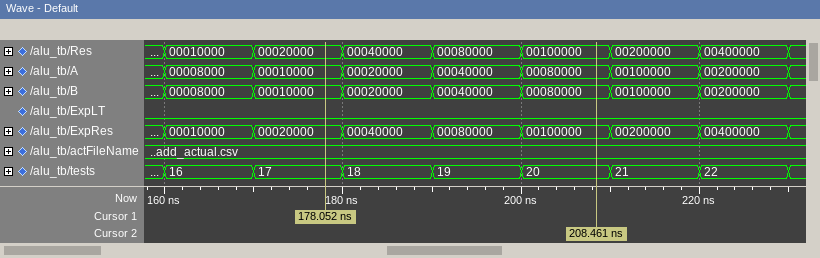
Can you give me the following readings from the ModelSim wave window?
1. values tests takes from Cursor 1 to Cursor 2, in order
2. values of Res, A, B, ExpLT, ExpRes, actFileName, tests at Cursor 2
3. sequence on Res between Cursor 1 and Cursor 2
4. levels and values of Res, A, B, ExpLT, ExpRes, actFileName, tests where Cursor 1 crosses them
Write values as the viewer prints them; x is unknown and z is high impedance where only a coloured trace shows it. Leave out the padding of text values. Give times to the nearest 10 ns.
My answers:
17, 18, 19, 20
Res=00100000, A=00080000, B=00080000, ExpLT=0, ExpRes=00100000, actFileName=add_actual.csv, tests=20
00020000, 00040000, 00080000, 00100000
Res=00020000, A=00010000, B=00010000, ExpLT=0, ExpRes=00020000, actFileName=add_actual.csv, tests=17
